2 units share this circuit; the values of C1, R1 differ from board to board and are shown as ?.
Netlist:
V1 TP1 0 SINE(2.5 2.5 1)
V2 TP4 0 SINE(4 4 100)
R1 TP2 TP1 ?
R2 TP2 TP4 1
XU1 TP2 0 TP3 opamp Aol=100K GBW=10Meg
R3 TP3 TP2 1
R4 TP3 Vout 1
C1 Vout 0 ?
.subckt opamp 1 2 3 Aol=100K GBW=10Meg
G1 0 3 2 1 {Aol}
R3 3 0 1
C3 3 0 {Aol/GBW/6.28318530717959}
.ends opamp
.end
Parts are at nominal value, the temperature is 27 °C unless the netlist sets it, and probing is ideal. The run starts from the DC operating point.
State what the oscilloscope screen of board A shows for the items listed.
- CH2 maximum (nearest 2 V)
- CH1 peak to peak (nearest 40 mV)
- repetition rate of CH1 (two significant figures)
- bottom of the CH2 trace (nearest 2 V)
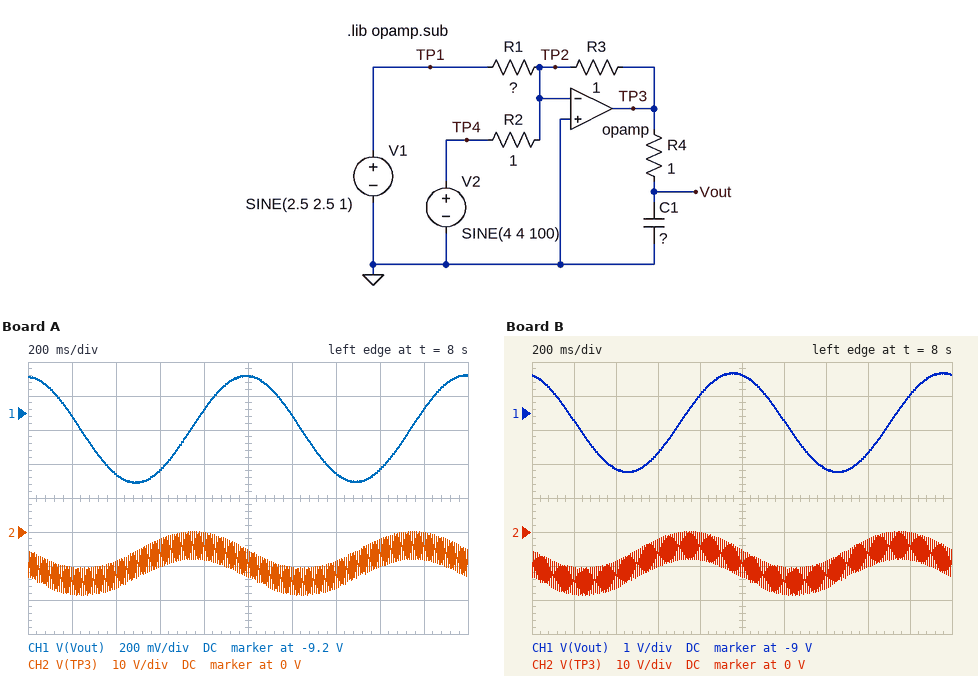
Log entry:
0 V
640 mV
1.0 Hz
-18 V
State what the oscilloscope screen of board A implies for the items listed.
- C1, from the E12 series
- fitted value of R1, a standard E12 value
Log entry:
2.7 F
0.47 Ω
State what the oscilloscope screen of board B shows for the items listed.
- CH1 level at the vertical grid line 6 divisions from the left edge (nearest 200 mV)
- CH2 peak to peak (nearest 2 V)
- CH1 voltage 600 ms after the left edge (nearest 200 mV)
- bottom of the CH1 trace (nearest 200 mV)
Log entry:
-9.2 V
18 V
-10.2 V
-10.8 V
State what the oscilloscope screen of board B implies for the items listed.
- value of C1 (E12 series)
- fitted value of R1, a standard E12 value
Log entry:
560 mF
0.47 Ω
